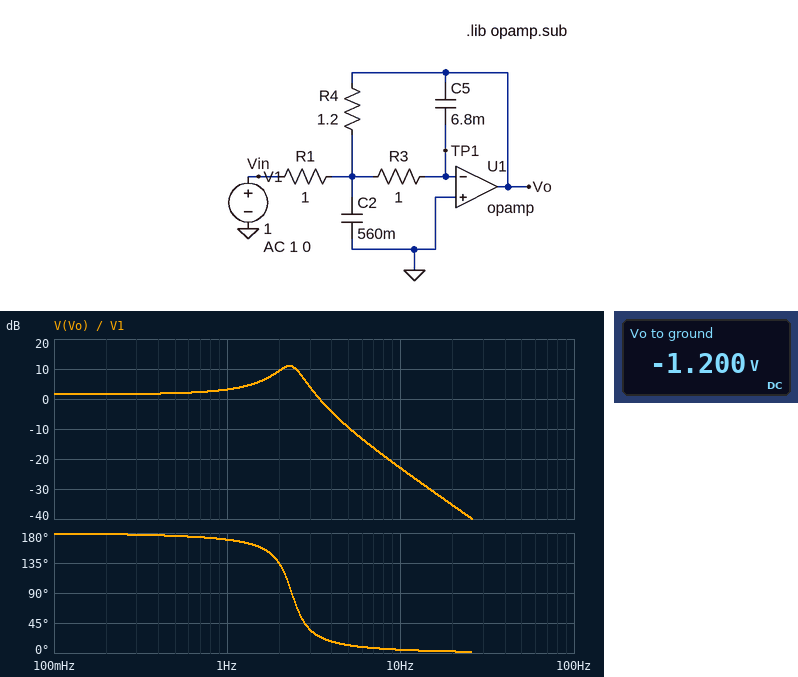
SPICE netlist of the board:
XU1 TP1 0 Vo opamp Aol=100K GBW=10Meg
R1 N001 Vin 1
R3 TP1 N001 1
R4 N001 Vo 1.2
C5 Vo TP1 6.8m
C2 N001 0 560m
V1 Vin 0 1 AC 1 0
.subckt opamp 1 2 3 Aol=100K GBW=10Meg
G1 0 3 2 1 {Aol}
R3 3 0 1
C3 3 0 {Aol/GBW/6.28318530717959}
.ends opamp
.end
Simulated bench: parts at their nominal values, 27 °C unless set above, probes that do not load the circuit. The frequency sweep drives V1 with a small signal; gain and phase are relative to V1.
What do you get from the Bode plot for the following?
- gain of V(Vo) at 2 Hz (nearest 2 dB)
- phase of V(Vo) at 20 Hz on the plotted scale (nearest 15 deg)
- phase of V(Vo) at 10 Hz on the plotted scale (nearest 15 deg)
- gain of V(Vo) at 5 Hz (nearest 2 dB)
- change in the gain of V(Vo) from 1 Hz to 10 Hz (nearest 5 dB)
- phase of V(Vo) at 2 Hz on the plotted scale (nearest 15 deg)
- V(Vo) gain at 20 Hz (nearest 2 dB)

10 dB
0 deg
0 deg
-10 dB
-25 dB
135 deg
-36 dB
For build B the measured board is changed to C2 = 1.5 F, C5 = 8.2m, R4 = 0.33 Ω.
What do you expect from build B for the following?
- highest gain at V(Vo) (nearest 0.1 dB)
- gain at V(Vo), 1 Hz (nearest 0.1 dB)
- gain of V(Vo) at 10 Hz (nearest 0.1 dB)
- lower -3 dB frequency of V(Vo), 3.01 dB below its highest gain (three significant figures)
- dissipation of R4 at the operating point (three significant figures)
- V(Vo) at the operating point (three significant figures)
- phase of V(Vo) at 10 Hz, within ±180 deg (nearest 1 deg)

3.8 dB
-8.2 dB
-33.2 dB
2.18 Hz
330 mW
-330 mV
3 deg
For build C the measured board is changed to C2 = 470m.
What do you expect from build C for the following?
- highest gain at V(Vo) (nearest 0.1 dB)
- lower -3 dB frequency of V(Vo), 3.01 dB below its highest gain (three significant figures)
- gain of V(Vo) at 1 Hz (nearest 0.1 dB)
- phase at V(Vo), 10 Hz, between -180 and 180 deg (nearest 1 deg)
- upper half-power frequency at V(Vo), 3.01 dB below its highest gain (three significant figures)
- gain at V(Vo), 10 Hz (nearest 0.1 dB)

10.3 dB
1.93 Hz
2.9 dB
6 deg
2.93 Hz
-21.5 dB
